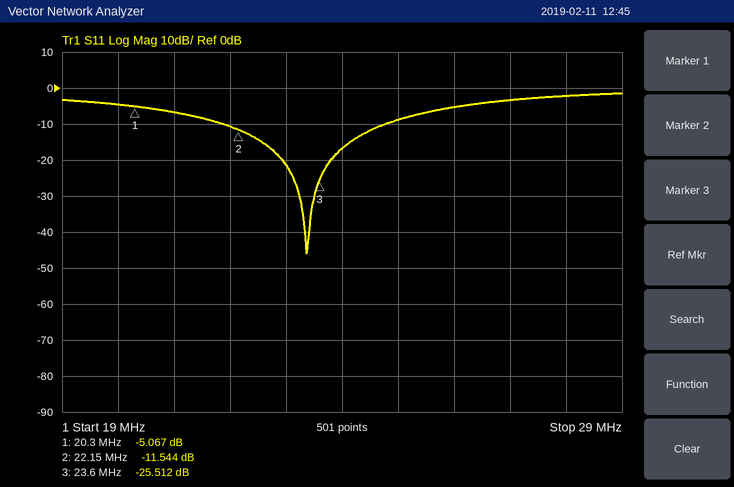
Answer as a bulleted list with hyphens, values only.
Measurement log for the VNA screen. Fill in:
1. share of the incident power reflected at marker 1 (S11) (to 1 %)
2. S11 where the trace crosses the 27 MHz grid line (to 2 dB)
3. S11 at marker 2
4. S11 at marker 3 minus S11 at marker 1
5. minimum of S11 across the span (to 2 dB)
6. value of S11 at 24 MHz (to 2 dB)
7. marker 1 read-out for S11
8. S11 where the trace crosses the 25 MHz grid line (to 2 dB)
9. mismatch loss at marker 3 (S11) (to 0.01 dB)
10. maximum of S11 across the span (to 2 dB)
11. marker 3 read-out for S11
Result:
- 31 %
- -4 dB
- -11.544 dB
- -20.445 dB
- -46 dB
- -16 dB
- -5.067 dB
- -8 dB
- 0.01 dB
- -2 dB
- -25.512 dB
